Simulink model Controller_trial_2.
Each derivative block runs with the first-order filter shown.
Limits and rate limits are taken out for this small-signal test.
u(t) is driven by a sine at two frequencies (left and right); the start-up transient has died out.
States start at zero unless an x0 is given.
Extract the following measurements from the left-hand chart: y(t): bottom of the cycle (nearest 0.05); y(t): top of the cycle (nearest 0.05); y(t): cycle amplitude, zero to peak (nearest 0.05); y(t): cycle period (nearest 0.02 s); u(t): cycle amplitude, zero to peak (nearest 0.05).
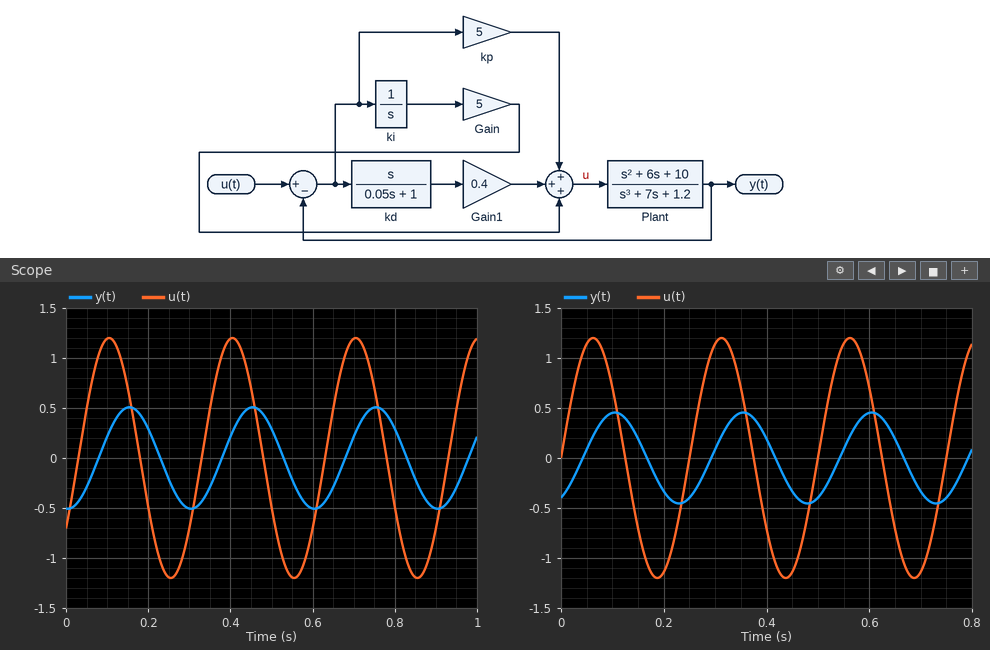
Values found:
-0.50
0.50
0.50
0.30 s
1.20
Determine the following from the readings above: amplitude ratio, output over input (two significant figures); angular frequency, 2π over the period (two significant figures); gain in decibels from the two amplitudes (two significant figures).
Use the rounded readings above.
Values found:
0.42
21 rad/s
-7.6 dB
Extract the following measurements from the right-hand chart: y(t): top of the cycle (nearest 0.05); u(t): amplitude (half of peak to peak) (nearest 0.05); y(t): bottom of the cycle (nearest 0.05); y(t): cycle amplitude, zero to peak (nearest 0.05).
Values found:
0.45
1.20
-0.45
0.45
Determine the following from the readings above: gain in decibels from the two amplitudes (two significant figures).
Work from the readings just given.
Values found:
-8.5 dB
